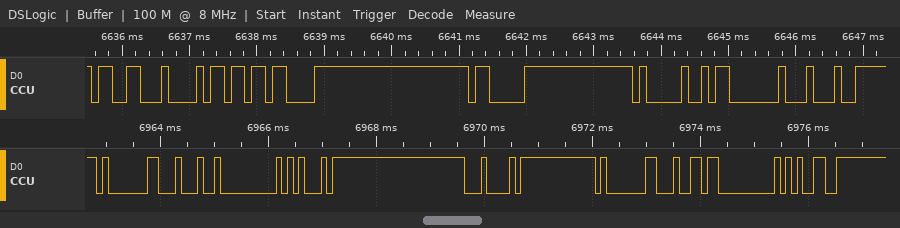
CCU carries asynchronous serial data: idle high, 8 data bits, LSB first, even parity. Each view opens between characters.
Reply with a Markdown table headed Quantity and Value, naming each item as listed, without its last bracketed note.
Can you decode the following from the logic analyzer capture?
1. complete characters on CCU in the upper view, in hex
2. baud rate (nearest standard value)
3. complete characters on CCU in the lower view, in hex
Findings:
| Quantity | Value |
|---|---|
| complete characters on CCU in the upper view, in hex | 33, 68, 1B, 83, 41, 03, 44 |
| baud rate | 9600 baud |
| complete characters on CCU in the lower view, in hex | 01, 44, 00, 45, 84, 01, 64, 00, 65 |
